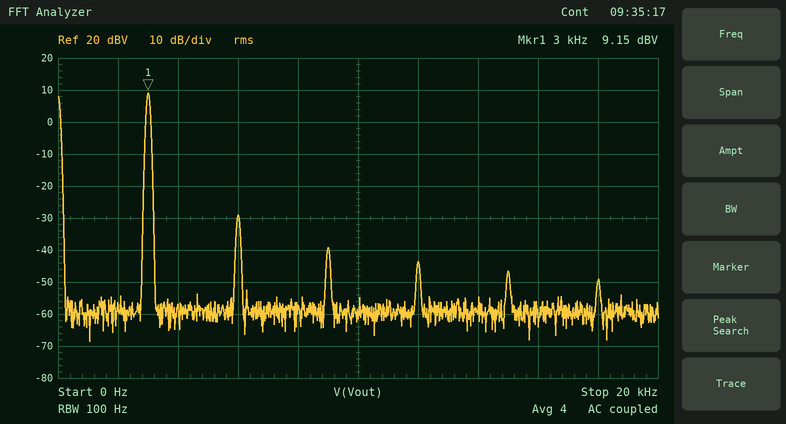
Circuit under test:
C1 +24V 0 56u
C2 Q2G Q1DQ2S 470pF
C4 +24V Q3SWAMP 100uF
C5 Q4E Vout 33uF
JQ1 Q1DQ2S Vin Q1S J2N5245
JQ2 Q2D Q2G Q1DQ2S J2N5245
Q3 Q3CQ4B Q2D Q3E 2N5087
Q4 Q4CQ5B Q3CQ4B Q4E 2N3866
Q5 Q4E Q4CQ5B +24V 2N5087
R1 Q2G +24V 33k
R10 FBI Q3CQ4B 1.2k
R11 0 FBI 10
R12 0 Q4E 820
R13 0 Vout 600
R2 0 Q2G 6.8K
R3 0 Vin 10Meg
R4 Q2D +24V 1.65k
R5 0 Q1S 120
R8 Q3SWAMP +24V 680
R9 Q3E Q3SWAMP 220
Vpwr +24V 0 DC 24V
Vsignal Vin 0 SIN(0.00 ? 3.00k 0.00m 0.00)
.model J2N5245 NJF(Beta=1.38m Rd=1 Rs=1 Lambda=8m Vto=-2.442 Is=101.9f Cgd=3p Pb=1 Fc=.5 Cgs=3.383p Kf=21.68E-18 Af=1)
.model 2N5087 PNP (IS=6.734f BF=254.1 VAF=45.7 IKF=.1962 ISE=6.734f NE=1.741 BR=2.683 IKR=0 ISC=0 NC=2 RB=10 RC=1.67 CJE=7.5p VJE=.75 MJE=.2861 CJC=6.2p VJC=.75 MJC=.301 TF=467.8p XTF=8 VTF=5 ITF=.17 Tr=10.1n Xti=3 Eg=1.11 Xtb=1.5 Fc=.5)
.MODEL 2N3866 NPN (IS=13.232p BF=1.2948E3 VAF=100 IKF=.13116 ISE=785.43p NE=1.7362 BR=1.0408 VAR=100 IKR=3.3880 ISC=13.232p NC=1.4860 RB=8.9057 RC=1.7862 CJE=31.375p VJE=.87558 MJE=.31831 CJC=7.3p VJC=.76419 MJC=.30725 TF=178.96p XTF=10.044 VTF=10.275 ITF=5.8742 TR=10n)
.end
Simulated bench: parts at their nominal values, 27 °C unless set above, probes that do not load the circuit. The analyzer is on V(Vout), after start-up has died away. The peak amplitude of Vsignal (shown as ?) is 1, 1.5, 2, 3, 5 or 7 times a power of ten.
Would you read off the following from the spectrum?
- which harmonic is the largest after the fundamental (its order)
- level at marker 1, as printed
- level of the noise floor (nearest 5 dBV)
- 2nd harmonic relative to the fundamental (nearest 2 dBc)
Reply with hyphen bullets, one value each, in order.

- 2
- 9.15 dBV
- -60 dBV
- -38 dBc
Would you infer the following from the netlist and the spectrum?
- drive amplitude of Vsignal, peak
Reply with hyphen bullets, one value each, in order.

- 150 mV
